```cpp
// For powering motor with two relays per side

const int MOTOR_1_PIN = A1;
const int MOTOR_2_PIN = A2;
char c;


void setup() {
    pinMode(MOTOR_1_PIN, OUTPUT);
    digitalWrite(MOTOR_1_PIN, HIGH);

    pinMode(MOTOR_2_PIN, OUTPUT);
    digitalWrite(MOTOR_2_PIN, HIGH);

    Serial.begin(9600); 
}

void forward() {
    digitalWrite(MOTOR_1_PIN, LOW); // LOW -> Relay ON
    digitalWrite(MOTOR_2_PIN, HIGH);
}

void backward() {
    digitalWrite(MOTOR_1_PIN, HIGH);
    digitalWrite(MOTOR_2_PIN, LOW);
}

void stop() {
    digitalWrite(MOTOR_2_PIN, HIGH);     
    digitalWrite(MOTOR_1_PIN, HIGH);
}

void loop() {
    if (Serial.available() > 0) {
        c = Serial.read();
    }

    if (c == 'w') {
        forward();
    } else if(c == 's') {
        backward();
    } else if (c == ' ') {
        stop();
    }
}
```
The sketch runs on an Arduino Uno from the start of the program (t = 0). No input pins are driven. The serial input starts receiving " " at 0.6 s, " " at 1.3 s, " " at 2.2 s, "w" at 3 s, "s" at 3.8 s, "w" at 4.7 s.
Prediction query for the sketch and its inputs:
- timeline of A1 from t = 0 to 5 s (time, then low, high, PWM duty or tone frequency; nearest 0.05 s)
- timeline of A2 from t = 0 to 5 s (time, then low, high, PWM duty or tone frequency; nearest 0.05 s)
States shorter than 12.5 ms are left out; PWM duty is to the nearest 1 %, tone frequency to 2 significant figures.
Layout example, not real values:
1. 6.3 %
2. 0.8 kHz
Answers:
1. 0 s high; 3 s low; 3.8 s high; 4.7 s low
2. 0 s high; 3.8 s low; 4.7 s high
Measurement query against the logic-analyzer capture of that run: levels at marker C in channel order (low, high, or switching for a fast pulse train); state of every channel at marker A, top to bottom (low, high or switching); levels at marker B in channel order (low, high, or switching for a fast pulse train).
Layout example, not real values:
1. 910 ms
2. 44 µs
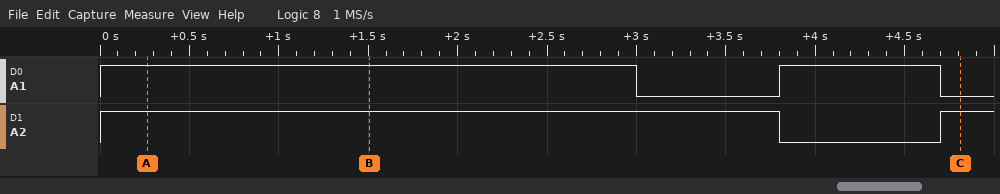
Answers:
1. A1 low, A2 high
2. A1 high, A2 high
3. A1 high, A2 high
